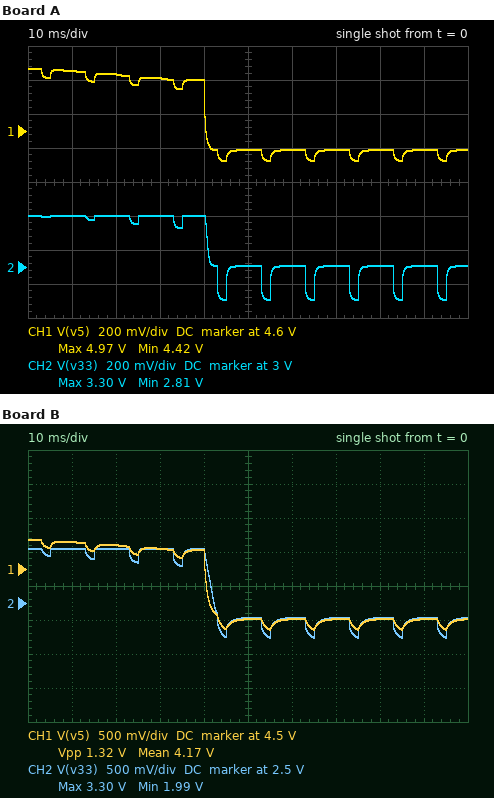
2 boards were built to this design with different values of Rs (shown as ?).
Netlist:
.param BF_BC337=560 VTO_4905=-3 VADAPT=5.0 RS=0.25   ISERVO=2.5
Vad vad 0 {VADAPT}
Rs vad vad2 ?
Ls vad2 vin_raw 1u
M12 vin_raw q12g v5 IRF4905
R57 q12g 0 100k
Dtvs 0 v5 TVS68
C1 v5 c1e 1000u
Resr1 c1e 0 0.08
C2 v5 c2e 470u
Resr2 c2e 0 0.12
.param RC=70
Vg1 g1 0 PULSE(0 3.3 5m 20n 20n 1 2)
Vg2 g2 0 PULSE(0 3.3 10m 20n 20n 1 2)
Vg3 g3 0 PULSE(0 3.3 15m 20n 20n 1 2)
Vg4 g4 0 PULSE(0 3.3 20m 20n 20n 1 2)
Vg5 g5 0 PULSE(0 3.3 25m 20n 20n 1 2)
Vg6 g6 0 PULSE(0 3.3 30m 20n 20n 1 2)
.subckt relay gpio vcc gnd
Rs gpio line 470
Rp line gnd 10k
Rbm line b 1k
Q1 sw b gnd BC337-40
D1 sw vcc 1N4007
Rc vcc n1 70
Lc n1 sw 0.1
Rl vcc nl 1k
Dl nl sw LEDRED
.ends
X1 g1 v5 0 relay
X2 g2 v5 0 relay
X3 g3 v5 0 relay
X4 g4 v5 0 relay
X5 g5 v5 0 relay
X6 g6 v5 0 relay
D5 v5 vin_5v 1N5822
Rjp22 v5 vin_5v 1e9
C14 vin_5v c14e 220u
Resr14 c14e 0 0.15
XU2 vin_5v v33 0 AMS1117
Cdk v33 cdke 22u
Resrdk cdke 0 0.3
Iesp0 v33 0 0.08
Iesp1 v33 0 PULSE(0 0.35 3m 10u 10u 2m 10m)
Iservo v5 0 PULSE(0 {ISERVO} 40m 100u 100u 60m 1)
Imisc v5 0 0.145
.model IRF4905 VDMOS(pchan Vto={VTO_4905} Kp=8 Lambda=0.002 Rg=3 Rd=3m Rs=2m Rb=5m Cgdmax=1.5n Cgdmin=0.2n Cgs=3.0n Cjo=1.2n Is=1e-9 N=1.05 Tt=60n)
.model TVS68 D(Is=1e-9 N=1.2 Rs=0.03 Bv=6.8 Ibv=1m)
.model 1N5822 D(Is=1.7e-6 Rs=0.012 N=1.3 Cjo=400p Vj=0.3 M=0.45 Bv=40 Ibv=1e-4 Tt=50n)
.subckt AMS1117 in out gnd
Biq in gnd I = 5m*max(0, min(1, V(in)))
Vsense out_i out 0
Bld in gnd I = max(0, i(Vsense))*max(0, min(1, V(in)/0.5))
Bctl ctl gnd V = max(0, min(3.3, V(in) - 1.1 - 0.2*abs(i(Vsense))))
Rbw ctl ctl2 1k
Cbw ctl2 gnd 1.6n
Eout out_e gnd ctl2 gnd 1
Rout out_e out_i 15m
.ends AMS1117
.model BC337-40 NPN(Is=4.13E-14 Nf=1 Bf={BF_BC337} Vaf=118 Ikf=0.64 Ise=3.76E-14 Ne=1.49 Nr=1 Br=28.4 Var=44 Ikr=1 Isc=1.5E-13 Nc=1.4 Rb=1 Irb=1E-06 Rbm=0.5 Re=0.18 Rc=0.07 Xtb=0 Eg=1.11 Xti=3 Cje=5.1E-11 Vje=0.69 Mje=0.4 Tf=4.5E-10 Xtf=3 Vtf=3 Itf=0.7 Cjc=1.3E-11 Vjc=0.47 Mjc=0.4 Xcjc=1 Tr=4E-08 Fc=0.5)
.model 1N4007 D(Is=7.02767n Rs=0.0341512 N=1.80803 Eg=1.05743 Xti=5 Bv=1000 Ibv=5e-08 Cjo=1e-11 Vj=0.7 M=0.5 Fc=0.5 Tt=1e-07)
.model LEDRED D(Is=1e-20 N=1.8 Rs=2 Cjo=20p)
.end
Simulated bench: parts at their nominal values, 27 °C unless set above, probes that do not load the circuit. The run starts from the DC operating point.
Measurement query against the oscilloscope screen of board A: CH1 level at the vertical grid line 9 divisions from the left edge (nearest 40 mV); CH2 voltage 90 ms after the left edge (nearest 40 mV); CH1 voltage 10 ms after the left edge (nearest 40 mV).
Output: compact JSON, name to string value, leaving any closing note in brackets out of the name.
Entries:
{"CH1 level at the vertical grid line 9 divisions from the left edge": "4.48 V", "CH2 voltage 90 ms after the left edge": "3.00 V", "CH1 voltage 10 ms after the left edge": "4.96 V"}
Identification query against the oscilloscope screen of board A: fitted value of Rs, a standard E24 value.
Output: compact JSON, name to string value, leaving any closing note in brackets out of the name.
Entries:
{"fitted value of Rs, a standard E24 value": "0.082 Ω"}
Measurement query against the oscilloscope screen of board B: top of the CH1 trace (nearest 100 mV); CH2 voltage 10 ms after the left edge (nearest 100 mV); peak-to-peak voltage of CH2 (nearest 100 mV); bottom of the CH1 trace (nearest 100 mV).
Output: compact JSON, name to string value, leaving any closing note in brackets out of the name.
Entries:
{"top of the CH1 trace": "4.9 V", "CH2 voltage 10 ms after the left edge": "3.3 V", "peak-to-peak voltage of CH2": "1.3 V", "bottom of the CH1 trace": "3.6 V"}
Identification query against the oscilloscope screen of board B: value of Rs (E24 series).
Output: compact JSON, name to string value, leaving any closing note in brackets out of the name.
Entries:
{"value of Rs": "0.27 Ω"}
